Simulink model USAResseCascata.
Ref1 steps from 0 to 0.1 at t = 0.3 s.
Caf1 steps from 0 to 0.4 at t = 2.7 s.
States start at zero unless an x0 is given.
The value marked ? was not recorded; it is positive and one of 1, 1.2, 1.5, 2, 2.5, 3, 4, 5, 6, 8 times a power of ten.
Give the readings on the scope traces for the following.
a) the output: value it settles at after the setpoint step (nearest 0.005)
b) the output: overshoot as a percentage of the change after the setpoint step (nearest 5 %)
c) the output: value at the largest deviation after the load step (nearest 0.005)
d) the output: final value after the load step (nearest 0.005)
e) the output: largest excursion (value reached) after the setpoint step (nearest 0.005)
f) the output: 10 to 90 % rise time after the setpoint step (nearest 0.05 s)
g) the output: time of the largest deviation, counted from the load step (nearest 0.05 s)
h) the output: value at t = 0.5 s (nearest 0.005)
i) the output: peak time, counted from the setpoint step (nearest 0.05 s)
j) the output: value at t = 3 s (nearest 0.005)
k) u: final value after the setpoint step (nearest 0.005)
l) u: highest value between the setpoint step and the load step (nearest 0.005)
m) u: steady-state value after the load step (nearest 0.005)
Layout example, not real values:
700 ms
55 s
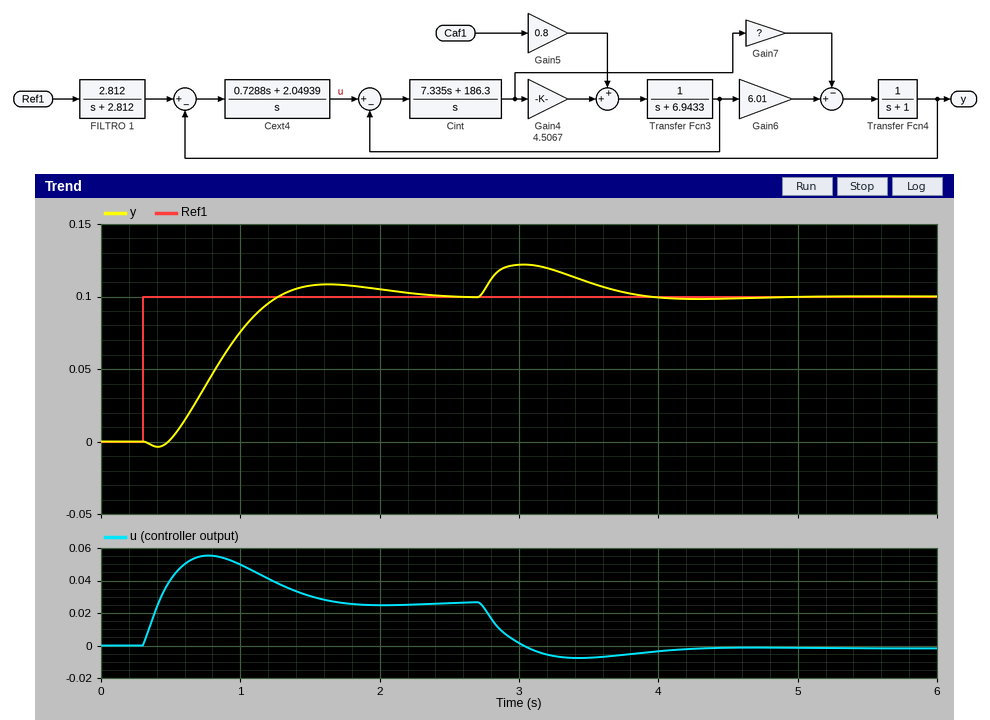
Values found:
0.100
10 %
0.120
0.100
0.110
0.55 s
0.35 s
0.000
1.35 s
0.120
0.025
0.055
0.000
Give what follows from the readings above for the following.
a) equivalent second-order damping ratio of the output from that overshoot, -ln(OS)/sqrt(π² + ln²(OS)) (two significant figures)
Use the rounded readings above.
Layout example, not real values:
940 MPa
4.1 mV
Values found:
0.59
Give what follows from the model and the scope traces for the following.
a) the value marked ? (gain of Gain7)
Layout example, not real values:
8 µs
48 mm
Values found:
1.5
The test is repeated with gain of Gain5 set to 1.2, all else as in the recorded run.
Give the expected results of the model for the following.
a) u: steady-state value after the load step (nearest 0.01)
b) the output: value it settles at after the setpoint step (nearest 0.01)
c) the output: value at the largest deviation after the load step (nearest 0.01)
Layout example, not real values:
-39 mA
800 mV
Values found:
-0.02
0.10
0.13
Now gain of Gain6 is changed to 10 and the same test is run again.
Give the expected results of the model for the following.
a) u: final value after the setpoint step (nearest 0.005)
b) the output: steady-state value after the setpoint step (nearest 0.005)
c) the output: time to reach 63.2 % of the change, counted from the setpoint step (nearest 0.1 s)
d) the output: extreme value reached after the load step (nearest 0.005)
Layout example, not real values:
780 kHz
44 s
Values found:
0.015
0.100
0.5 s
0.115
